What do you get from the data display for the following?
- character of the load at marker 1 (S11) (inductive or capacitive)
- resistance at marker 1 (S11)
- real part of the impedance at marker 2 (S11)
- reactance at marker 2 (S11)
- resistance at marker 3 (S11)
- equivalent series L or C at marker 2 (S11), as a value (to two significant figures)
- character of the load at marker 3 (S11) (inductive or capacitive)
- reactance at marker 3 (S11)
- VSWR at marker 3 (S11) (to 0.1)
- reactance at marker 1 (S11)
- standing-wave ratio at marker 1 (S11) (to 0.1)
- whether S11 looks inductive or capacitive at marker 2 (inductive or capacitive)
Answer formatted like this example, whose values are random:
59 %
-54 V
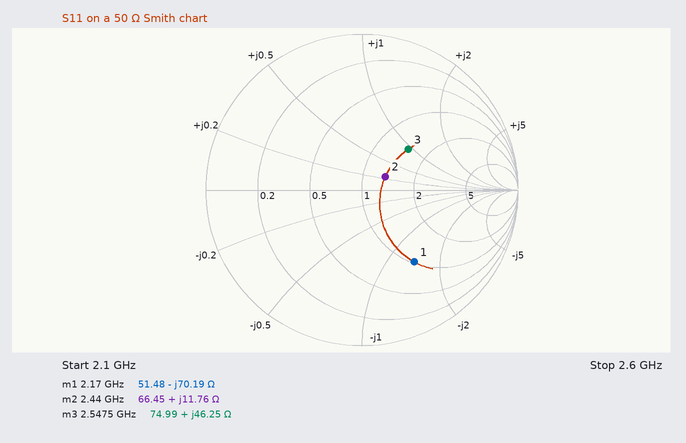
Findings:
capacitive
51.48 Ω
66.45 Ω
+11.76 Ω
74.99 Ω
770 pH
inductive
+46.25 Ω
2.3
-70.19 Ω
3.6
inductive
